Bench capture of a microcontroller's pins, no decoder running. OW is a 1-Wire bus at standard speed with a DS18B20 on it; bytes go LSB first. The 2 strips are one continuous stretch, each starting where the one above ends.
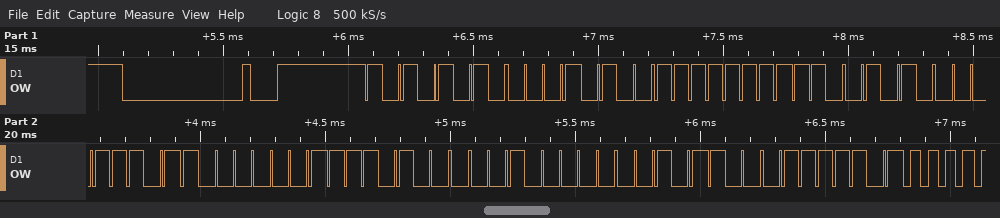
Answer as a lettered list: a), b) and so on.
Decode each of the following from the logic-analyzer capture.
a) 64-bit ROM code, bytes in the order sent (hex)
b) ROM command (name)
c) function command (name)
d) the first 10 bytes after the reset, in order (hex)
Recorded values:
a) 28 FF 53 B8 81 17 04 34
b) Match ROM
c) Read Scratchpad
d) 55 28 FF 53 B8 81 17 04 34 BE
